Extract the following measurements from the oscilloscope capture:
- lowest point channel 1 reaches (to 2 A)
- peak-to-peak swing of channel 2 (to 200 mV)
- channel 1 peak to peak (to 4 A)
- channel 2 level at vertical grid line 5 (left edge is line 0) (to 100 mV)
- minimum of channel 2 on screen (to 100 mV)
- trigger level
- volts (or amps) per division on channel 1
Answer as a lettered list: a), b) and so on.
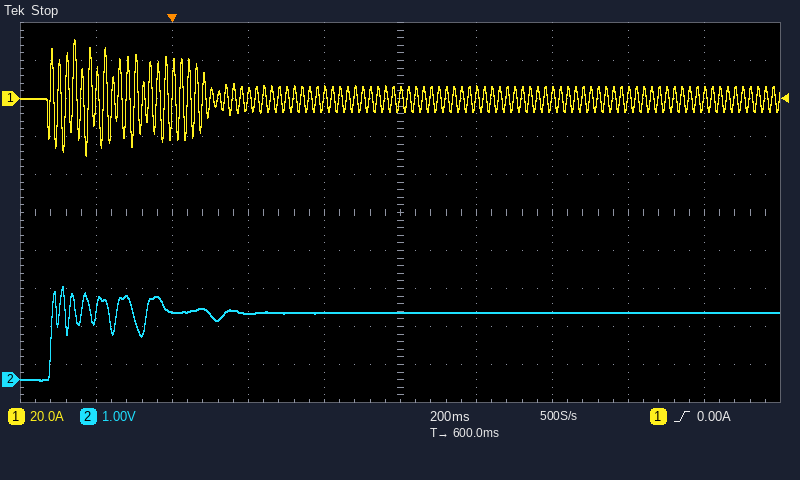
a) -30 A
b) 2.4 V
c) 60 A
d) 1.8 V
e) 0.0 V
f) 0.00 A
g) 20 A
